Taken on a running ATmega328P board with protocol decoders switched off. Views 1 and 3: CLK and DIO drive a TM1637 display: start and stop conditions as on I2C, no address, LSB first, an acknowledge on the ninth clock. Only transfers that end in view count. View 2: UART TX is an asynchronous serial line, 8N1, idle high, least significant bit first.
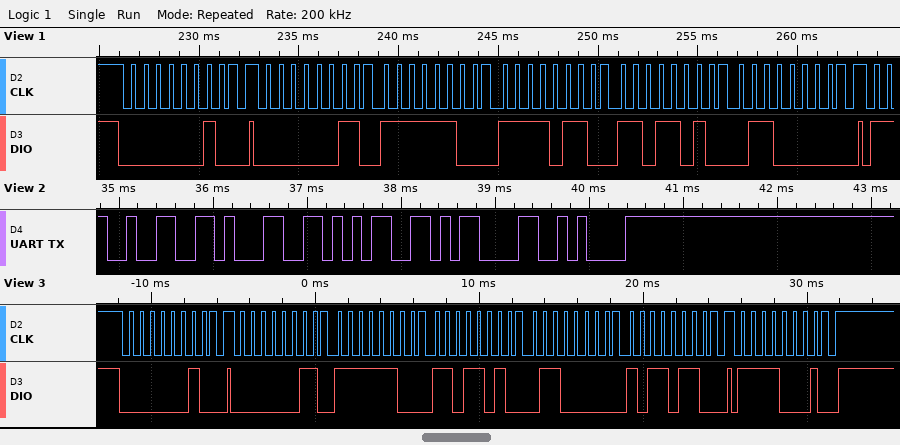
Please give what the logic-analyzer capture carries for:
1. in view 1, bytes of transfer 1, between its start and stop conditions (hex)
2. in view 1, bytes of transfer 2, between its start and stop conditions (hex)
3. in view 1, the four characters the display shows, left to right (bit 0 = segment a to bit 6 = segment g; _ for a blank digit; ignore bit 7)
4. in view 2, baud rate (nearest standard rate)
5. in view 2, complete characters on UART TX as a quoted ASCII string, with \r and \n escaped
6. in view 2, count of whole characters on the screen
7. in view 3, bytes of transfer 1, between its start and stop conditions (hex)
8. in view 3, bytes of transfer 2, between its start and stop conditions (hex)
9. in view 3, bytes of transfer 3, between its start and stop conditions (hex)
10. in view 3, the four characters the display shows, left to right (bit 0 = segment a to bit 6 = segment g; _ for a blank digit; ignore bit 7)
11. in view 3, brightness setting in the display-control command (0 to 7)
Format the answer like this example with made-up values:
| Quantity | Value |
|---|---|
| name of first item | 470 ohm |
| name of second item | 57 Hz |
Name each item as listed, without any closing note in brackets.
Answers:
| Quantity | Value |
|---|---|
| in view 1, bytes of transfer 1, between its start and stop conditions | 40 |
| in view 1, bytes of transfer 2, between its start and stop conditions | C0 3F 6F 5B 06 |
| in view 1, the four characters the display shows, left to right | 0921 |
| in view 2, baud rate | 9600 baud |
| in view 2, complete characters on UART TX as a quoted ASCII string, with \r and \n escaped | "215\r\n" |
| in view 2, count of whole characters on the screen | 5 |
| in view 3, bytes of transfer 1, between its start and stop conditions | 40 |
| in view 3, bytes of transfer 2, between its start and stop conditions | C0 3F 5B 06 6D |
| in view 3, bytes of transfer 3, between its start and stop conditions | 8F |
| in view 3, the four characters the display shows, left to right | 0215 |
| in view 3, brightness setting in the display-control command | 7 |
